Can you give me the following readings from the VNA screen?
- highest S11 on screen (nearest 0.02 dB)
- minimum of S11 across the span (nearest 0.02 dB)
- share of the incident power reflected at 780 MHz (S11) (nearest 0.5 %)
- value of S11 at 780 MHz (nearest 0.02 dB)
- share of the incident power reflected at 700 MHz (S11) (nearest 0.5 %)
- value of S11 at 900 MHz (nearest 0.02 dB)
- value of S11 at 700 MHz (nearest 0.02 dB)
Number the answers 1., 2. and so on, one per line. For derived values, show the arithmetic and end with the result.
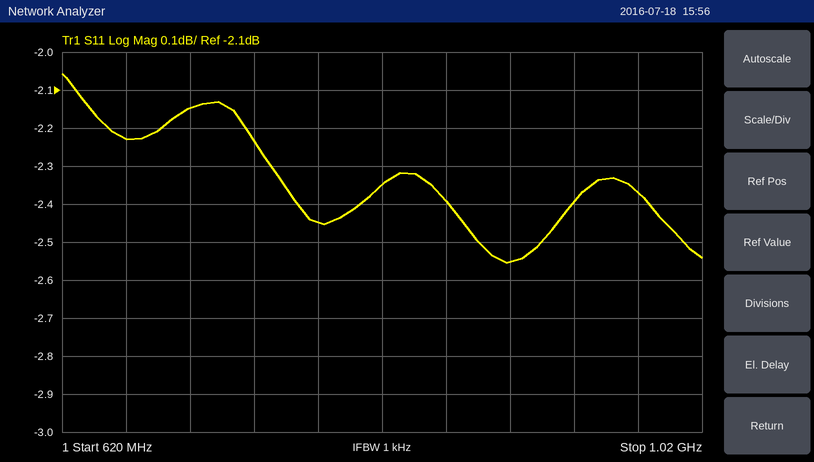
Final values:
1. -2.06 dB
2. -2.56 dB
3. 10^(-2.44/10) ≈ 57.0 %
4. -2.44 dB
5. 10^(-2.14/10) ≈ 61.1 %, so 61.0 % to the nearest 0.5 %
6. -2.56 dB
7. -2.14 dB
